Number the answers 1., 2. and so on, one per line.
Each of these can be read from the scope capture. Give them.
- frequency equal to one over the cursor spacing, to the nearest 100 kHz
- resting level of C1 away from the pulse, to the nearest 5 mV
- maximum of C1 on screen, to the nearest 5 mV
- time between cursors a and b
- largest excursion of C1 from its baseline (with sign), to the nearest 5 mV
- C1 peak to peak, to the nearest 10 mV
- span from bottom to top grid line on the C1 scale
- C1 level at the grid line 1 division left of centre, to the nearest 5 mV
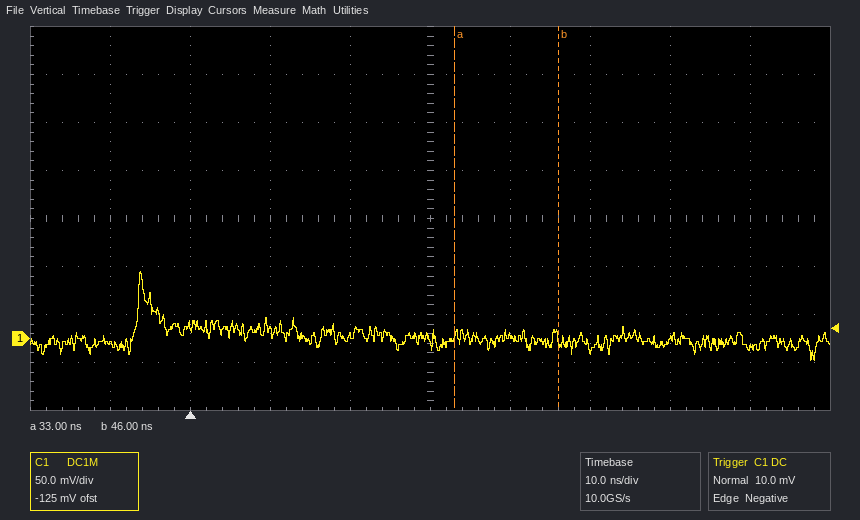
1. 76.9 MHz
2. 0 mV
3. 70 mV
4. 13 ns
5. +70 mV
6. 90 mV
7. 400 mV
8. 0 mV
